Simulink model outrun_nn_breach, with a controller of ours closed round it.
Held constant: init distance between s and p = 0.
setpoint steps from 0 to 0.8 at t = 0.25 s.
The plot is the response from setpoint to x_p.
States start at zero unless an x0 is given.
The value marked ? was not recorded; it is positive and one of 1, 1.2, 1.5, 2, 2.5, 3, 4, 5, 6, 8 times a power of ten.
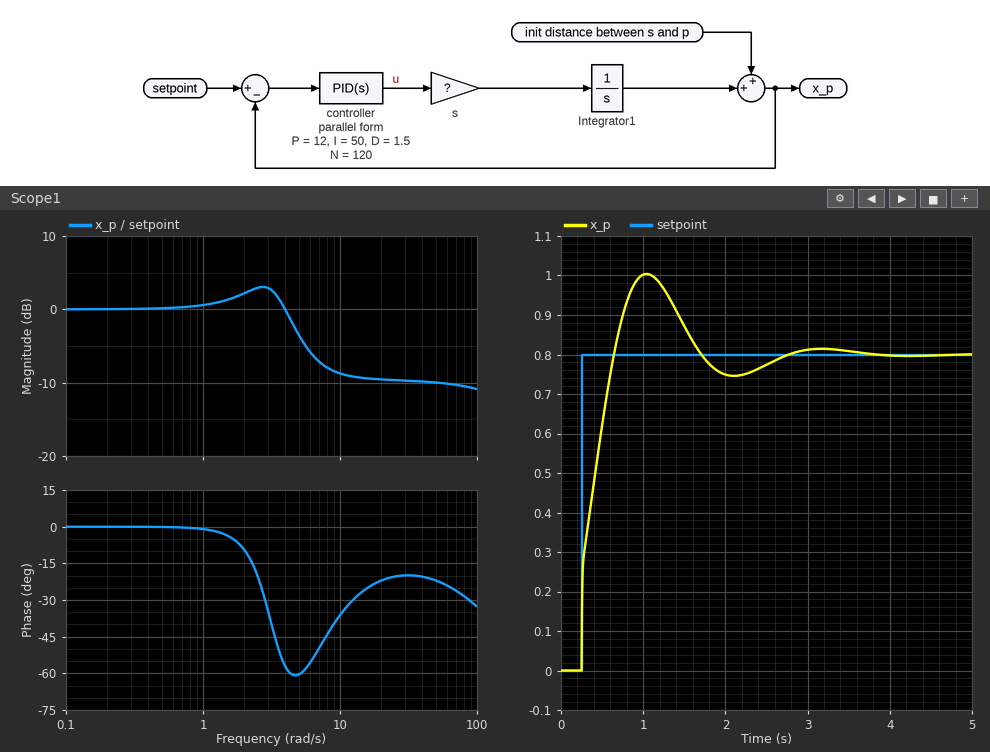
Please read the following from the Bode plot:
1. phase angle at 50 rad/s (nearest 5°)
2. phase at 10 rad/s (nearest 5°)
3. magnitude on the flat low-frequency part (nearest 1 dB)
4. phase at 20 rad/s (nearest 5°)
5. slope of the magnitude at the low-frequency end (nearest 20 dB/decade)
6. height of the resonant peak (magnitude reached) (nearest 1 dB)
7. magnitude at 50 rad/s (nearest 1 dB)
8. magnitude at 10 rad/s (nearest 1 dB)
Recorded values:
-20°
-35°
0 dB
-20°
0 dB/decade
3 dB
-10 dB
-9 dB
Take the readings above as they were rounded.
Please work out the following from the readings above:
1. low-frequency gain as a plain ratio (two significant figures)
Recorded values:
1.0
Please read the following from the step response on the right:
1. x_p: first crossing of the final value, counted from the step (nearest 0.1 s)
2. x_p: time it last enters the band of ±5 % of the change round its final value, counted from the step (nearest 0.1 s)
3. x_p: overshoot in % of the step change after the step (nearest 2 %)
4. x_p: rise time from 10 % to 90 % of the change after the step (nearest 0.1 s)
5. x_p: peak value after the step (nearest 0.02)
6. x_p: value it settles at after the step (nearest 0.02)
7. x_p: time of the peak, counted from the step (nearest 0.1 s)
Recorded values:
0.4 s
2.1 s
26 %
0.3 s
1.00
0.80
0.8 s
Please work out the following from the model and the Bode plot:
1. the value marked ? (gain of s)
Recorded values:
0.3
